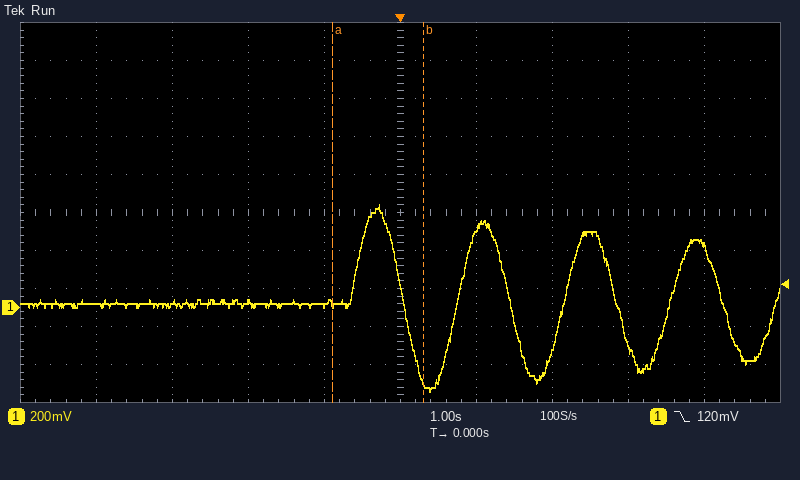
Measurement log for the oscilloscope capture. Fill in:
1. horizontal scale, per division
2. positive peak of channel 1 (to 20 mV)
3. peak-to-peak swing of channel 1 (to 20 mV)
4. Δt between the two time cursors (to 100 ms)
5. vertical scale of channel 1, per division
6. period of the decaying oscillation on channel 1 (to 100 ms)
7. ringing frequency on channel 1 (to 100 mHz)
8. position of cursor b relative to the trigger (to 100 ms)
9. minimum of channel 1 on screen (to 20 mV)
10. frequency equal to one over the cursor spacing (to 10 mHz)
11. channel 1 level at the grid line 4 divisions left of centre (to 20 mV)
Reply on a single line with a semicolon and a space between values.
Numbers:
1 s; 540 mV; 980 mV; 1.2 s; 200 mV; 1.4 s; 700 mHz; +300 ms; -440 mV; 830 mHz; 20 mV
